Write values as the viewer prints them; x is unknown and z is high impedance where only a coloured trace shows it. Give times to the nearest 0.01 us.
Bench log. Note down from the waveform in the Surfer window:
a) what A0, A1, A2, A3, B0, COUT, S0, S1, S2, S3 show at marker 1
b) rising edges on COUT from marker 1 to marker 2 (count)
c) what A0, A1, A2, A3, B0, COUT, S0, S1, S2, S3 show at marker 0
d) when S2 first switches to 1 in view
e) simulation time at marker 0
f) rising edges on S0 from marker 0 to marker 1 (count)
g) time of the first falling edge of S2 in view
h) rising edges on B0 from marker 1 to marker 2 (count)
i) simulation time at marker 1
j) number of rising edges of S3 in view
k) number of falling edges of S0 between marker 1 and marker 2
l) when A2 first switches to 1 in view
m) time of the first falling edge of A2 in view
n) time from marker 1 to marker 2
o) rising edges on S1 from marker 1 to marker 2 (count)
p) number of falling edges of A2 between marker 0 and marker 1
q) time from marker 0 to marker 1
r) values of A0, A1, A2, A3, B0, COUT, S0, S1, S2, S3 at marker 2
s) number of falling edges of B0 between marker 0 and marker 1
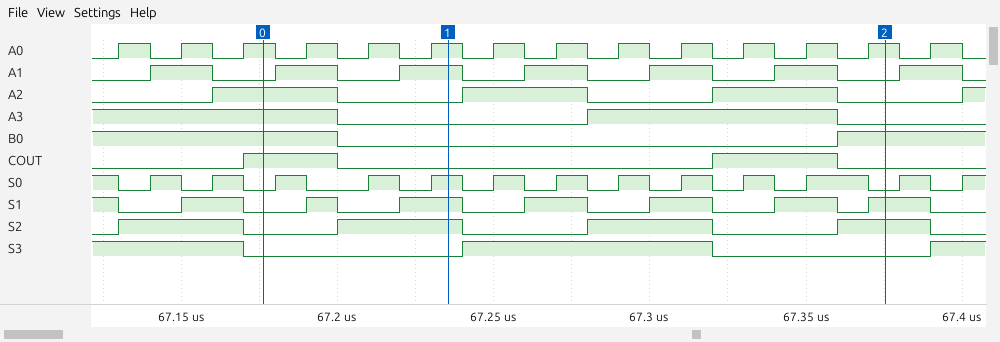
A0=1, A1=1, A2=0, A3=0, B0=0, COUT=0, S0=1, S1=1, S2=1, S3=0
1
A0=1, A1=0, A2=1, A3=1, B0=1, COUT=1, S0=0, S1=0, S2=0, S3=0
67.13 us
67.18 us
3
67.17 us
1
67.24 us
2
7
67.16 us
67.2 us
0.14 us
4
1
0.06 us
A0=1, A1=0, A2=0, A3=0, B0=1, COUT=0, S0=0, S1=1, S2=1, S3=0
1
